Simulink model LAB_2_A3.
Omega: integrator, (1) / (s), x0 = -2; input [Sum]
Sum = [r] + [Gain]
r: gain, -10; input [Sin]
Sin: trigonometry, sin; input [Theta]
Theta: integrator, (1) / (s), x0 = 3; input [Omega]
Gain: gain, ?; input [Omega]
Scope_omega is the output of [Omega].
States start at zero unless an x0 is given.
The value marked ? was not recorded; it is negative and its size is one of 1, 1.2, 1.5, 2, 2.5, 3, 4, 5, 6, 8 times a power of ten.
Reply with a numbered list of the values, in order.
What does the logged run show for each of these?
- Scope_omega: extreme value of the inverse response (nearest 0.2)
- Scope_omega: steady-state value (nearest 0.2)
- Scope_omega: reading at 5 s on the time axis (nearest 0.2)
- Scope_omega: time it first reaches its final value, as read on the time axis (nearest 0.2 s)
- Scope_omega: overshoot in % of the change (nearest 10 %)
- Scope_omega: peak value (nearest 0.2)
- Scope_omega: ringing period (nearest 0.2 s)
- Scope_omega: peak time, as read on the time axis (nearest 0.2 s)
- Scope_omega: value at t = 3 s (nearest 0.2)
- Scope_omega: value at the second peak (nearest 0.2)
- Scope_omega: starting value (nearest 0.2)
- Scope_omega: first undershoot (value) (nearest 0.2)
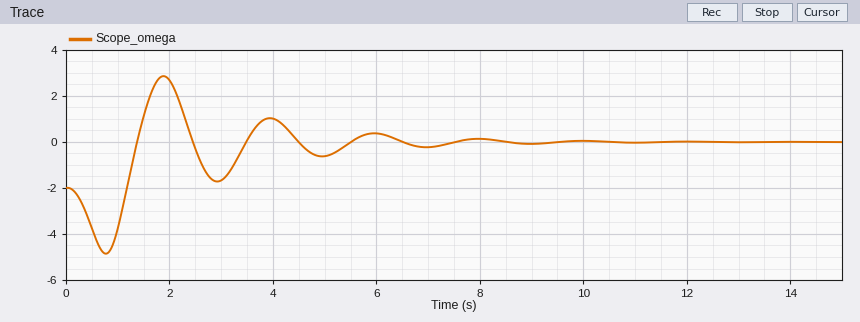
1. -4.8
2. 0.0
3. -0.6
4. 1.4 s
5. 140 %
6. 2.8
7. 2.0 s
8. 1.8 s
9. -1.6
10. 1.0
11. -2.0
12. -1.8
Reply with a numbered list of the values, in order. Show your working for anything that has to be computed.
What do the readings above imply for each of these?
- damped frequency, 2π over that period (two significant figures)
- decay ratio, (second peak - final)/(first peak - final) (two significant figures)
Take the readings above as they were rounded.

1. 2π / 2 = 3.1 rad/s
2. (1 - 0) / (2.8 - 0) = 0.36
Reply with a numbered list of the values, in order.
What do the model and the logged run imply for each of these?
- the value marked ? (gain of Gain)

1. -1
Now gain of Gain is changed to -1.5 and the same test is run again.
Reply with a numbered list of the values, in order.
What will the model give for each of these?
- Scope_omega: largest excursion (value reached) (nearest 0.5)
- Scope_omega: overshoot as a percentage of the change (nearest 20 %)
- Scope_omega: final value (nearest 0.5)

1. 2.0
2. 100 %
3. 0.0
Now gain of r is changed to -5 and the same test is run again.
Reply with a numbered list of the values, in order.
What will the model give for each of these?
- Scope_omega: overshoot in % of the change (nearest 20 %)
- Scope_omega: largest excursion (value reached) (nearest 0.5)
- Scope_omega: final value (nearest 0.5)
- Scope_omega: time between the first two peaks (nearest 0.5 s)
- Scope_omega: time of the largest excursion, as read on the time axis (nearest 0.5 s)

1. 80 %
2. 1.5
3. 0.0
4. 3.0 s
5. 2.5 s
